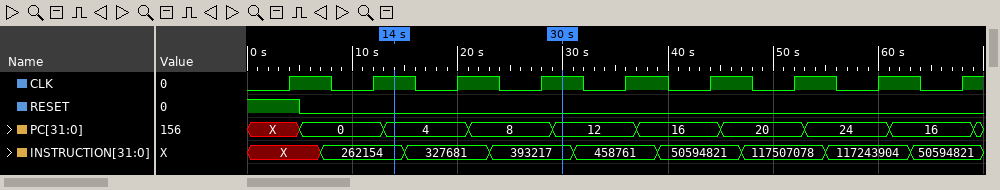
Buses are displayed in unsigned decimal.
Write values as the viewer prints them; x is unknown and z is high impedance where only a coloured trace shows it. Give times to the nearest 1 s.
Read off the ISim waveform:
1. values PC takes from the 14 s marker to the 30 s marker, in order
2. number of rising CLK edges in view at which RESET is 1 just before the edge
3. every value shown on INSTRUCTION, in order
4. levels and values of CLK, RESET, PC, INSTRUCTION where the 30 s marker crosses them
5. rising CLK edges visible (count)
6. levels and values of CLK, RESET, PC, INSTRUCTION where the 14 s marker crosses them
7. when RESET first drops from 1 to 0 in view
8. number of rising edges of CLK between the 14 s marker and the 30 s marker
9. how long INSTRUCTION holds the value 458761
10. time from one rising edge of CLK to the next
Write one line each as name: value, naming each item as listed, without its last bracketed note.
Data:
values PC takes from the 14 s marker to the 30 s marker, in order: 4, 8, 12
number of rising CLK edges in view at which RESET is 1 just before the edge: 1
every value shown on INSTRUCTION, in order: X, 262154, 327681, 393217, 458761, 50594821, 117507078, 117243904, 50594821
levels and values of CLK, RESET, PC, INSTRUCTION where the 30 s marker crosses them: CLK=1, RESET=0, PC=12, INSTRUCTION=393217
rising CLK edges visible: 9
levels and values of CLK, RESET, PC, INSTRUCTION where the 14 s marker crosses them: CLK=1, RESET=0, PC=4, INSTRUCTION=262154
when RESET first drops from 1 to 0 in view: 5 s
number of rising edges of CLK between the 14 s marker and the 30 s marker: 2
how long INSTRUCTION holds the value 458761: 8 s
time from one rising edge of CLK to the next: 8 s
